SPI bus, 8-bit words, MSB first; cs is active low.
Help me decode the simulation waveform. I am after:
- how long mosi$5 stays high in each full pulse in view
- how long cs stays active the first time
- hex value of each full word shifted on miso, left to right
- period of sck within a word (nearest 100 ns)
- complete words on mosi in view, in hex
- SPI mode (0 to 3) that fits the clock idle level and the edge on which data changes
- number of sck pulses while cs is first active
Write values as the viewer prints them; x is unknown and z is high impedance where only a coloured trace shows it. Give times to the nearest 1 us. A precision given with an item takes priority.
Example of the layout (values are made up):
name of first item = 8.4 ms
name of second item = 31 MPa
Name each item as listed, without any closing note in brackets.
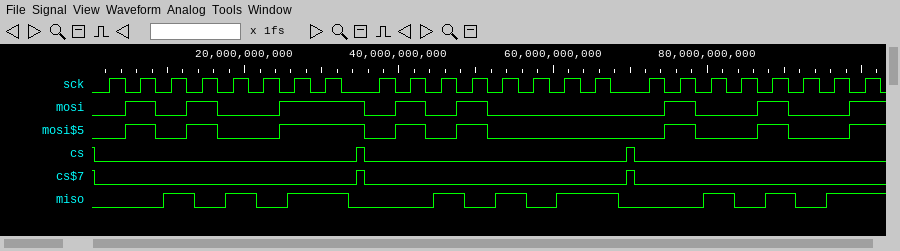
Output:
how long mosi$5 stays high in each full pulse in view = 4 us, 4 us, 11 us, 4 us, 4 us, 4 us, 4 us
how long cs stays active the first time = 34 us
hex value of each full word shifted on miso, left to right = 2B, 2B, 2B
period of sck within a word = 4000 ns
complete words on mosi in view, in hex = 53, 50, 49
SPI mode (0 to 3) that fits the clock idle level and the edge on which data changes = 0
number of sck pulses while cs is first active = 8
